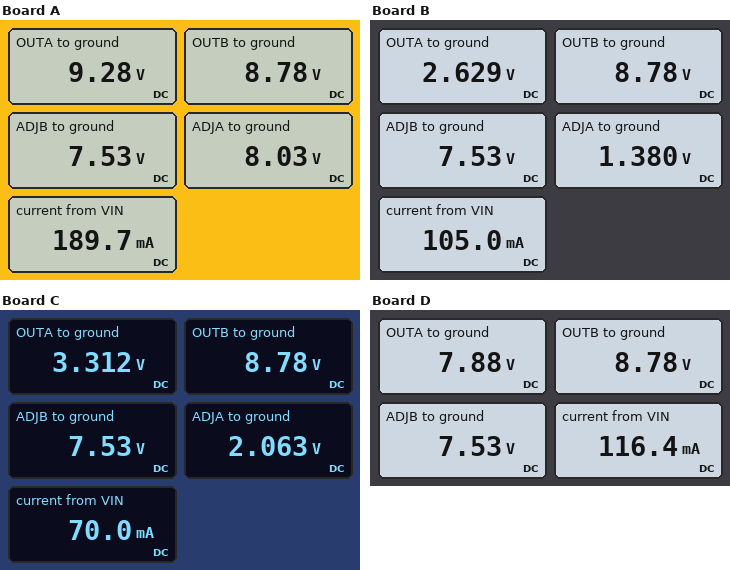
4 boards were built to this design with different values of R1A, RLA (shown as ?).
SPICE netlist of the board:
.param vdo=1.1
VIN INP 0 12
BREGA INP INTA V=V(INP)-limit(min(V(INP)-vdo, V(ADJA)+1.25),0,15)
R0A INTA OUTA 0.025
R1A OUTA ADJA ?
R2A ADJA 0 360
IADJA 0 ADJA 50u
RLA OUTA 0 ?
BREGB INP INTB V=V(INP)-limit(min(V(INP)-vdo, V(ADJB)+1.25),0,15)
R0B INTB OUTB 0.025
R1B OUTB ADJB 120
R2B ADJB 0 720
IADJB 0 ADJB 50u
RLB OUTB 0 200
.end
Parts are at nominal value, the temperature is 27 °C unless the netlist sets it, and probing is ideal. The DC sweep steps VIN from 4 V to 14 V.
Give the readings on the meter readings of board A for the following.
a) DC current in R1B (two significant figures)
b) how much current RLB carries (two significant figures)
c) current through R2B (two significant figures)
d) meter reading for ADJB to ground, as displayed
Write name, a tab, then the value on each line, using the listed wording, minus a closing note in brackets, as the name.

DC current in R1B	10 mA
how much current RLB carries	44 mA
current through R2B	10 mA
meter reading for ADJB to ground, as displayed	7.53 V
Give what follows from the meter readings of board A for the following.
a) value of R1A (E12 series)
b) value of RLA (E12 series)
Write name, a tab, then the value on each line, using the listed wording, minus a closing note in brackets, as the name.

value of R1A	56 Ω
value of RLA	82 Ω
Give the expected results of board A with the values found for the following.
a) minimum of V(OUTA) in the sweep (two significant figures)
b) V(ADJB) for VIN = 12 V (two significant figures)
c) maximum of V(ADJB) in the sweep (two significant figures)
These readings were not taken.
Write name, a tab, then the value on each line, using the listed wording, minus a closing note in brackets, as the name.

minimum of V(OUTA) in the sweep	2.9 V
V(ADJB) for VIN = 12 V	7.5 V
maximum of V(ADJB) in the sweep	7.5 V
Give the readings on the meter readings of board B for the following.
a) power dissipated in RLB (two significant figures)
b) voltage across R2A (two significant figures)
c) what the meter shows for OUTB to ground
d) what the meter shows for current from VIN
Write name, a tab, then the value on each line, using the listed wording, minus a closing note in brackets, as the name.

power dissipated in RLB	390 mW
voltage across R2A	1.4 V
what the meter shows for OUTB to ground	8.78 V
what the meter shows for current from VIN	105.0 mA
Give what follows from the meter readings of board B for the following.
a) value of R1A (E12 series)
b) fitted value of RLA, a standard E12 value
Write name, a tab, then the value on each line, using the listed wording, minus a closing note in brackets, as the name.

value of R1A	330 Ω
fitted value of RLA, a standard E12 value	56 Ω
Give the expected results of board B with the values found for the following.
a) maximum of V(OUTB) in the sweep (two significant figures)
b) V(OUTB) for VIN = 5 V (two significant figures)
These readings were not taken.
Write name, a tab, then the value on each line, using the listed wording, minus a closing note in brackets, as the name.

maximum of V(OUTB) in the sweep	8.8 V
V(OUTB) for VIN = 5 V	3.9 V
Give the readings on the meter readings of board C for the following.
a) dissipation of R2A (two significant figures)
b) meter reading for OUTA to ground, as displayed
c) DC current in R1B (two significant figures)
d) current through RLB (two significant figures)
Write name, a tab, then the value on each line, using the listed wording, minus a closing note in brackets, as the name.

dissipation of R2A	12 mW
meter reading for OUTA to ground, as displayed	3.312 V
DC current in R1B	10 mA
current through RLB	44 mA
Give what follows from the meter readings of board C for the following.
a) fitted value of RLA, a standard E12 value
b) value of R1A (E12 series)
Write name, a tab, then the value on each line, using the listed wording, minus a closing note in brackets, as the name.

fitted value of RLA, a standard E12 value	330 Ω
value of R1A	220 Ω
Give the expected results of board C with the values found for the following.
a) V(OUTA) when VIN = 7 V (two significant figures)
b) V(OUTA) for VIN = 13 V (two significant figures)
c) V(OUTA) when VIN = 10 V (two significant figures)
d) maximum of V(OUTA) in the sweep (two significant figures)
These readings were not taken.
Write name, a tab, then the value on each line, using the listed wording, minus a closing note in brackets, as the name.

V(OUTA) when VIN = 7 V	3.3 V
V(OUTA) for VIN = 13 V	3.3 V
V(OUTA) when VIN = 10 V	3.3 V
maximum of V(OUTA) in the sweep	3.3 V
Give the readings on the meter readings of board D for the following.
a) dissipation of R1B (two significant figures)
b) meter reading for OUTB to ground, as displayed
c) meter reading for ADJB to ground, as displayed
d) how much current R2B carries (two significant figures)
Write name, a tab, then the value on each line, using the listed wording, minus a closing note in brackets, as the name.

dissipation of R1B	13 mW
meter reading for OUTB to ground, as displayed	8.78 V
meter reading for ADJB to ground, as displayed	7.53 V
how much current R2B carries	10 mA
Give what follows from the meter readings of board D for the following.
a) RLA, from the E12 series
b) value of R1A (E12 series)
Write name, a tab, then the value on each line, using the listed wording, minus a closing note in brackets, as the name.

RLA, from the E12 series	180 Ω
value of R1A	68 Ω
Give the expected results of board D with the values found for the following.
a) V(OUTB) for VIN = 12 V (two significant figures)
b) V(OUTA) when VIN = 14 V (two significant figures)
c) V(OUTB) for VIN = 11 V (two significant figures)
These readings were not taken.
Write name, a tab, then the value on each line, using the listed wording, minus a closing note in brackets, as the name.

V(OUTB) for VIN = 12 V	8.8 V
V(OUTA) when VIN = 14 V	7.9 V
V(OUTB) for VIN = 11 V	8.8 V
